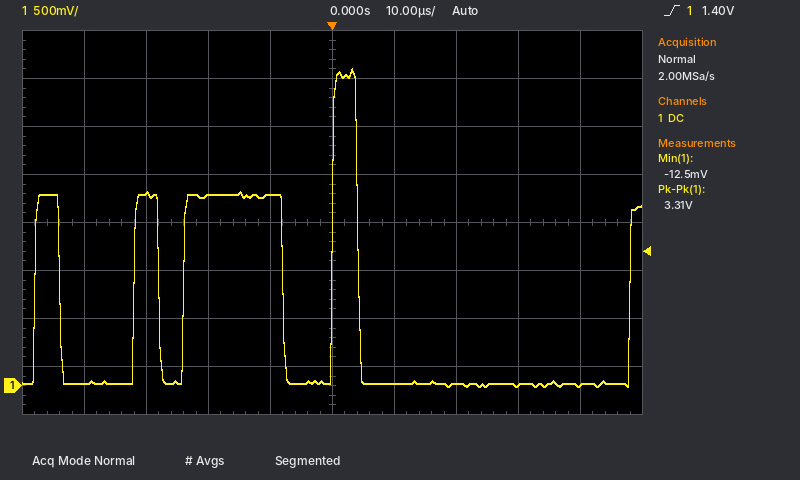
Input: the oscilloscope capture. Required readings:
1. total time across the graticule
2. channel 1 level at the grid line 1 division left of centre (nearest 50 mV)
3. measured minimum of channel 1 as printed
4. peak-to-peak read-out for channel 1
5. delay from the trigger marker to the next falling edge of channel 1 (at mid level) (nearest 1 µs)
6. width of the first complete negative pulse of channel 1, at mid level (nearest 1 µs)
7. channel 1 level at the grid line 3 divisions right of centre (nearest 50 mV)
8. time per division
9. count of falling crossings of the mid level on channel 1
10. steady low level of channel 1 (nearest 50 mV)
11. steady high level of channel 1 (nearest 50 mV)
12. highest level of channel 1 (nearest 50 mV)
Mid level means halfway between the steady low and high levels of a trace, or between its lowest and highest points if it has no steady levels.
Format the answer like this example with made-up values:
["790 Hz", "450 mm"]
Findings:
["100 µs", "2.00 V", "-12.5 mV", "3.31 V", "4 µs", "12 µs", "0 mV", "10 µs", "4", "0 mV", "2.00 V", "3.30 V"]
